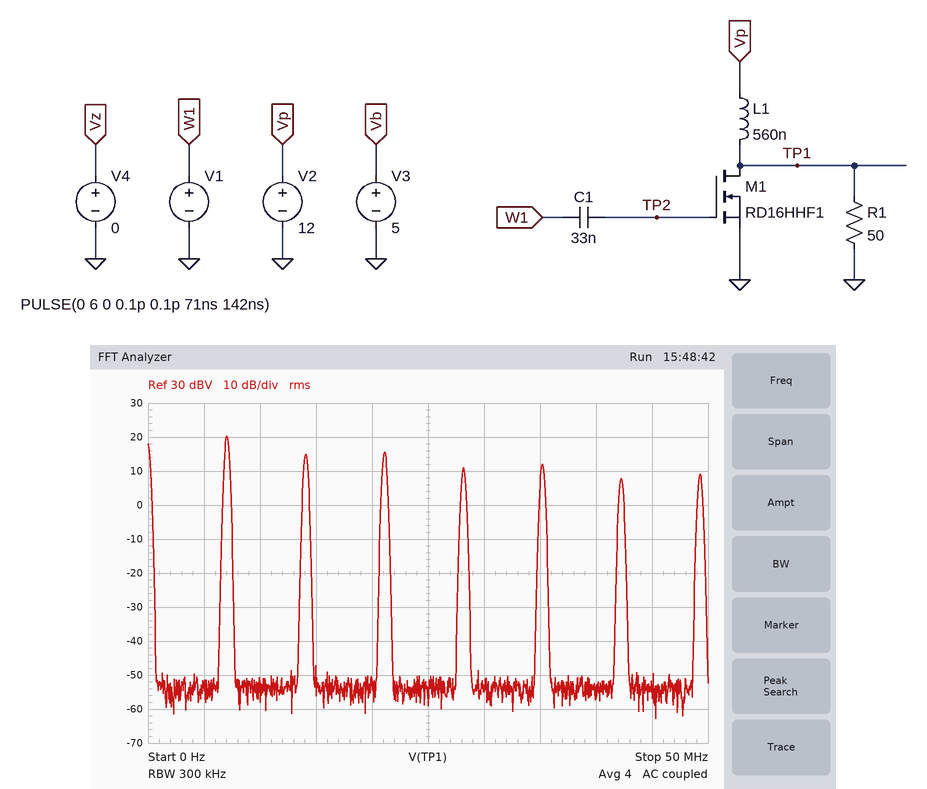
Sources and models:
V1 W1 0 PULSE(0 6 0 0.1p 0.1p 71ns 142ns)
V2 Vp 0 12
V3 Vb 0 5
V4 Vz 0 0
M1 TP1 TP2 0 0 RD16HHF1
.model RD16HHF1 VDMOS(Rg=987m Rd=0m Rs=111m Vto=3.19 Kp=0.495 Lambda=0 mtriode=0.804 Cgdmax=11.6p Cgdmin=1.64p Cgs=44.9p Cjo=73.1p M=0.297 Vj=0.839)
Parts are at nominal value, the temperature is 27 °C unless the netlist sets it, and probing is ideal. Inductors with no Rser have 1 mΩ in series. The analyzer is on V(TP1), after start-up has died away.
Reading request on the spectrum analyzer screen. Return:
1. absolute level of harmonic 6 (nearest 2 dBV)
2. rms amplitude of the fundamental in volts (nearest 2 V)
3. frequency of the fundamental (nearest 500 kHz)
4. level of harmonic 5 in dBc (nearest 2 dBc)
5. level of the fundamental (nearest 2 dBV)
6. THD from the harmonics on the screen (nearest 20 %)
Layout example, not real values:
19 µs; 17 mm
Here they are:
8 dBV; 10 V; 7.0 MHz; -8 dBc; 20 dBV; 100 %
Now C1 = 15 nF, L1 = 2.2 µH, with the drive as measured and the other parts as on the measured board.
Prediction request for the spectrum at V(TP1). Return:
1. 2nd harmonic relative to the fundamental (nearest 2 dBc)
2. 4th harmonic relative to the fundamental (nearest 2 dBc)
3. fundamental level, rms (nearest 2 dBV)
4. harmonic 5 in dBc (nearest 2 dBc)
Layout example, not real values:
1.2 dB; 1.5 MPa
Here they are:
-14 dBc; -20 dBc; 20 dBV; -14 dBc
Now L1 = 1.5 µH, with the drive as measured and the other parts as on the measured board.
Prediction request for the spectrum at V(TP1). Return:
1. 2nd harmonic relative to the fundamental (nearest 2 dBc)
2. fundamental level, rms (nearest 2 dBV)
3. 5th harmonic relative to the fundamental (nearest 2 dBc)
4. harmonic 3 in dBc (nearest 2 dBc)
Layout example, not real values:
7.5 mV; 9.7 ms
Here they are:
-12 dBc; 20 dBV; -12 dBc; -8 dBc
